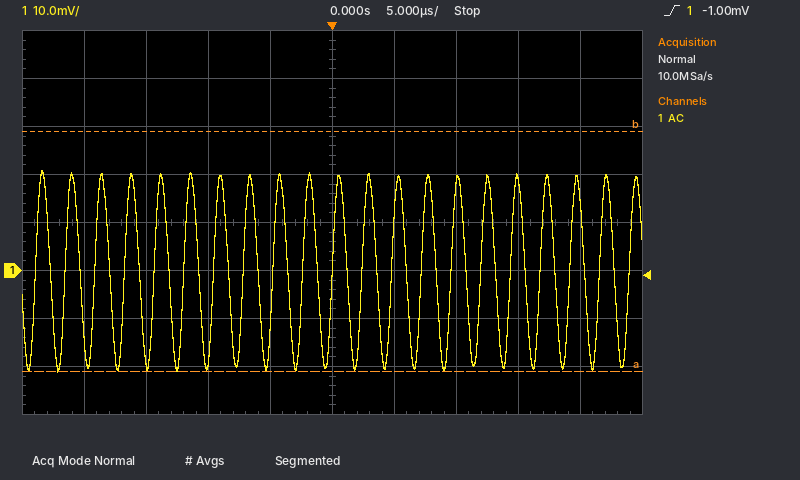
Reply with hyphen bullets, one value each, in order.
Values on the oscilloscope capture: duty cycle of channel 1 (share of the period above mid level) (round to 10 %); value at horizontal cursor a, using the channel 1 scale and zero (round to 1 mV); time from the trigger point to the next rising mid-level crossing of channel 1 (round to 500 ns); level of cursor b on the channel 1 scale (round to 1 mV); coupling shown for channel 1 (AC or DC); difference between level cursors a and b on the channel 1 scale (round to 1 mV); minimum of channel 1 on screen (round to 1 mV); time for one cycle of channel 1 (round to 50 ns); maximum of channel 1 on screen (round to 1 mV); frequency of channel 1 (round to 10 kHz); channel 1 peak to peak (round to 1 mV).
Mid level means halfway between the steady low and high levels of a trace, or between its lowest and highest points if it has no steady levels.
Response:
- 50 %
- -21 mV
- 2.5 µs
- 29 mV
- AC
- 50 mV
- -21 mV
- 2.40 µs
- 21 mV
- 420 kHz
- 42 mV
